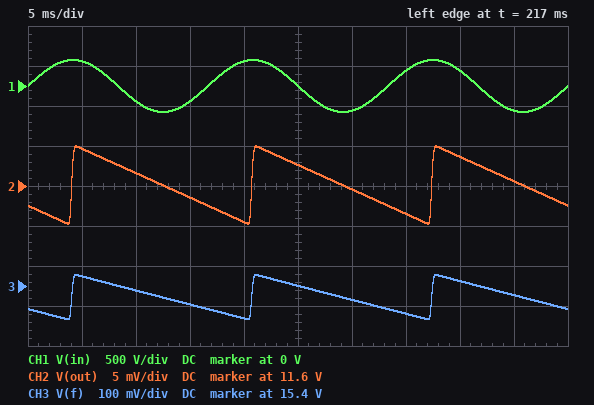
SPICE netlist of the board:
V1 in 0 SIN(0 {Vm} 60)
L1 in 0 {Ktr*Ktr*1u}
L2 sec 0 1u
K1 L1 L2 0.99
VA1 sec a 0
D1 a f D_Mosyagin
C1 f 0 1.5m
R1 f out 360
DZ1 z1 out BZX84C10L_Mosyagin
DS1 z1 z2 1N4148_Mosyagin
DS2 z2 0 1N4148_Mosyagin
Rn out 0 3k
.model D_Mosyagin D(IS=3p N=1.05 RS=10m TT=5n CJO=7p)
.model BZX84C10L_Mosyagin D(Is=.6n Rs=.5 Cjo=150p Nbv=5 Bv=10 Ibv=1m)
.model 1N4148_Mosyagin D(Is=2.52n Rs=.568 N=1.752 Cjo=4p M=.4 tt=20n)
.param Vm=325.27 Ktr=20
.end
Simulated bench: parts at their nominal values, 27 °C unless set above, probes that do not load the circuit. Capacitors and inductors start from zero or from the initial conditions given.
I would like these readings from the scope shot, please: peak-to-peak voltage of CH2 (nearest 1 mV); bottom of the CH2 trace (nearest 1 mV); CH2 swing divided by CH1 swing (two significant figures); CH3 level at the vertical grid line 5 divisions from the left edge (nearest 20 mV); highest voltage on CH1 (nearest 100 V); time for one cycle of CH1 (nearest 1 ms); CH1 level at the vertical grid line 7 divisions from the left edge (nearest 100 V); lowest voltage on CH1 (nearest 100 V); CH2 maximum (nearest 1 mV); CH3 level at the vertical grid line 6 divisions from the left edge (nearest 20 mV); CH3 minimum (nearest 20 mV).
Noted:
10 mV
11.590 V
0.000015
15.40 V
300 V
17 ms
200 V
-300 V
11.600 V
15.36 V
15.32 V
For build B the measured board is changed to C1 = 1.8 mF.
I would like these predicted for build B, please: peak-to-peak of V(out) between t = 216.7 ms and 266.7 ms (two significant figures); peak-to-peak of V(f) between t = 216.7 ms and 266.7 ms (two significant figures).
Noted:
8.1 mV
93 mV
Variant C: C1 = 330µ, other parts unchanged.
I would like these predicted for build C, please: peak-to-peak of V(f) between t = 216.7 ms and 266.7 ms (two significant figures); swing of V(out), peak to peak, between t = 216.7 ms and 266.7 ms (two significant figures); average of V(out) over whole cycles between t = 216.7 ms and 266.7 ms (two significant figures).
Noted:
480 mV
44 mV
12 V
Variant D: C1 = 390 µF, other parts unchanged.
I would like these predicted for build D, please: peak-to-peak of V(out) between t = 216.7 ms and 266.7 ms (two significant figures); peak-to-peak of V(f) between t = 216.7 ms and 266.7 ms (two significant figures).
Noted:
37 mV
410 mV
